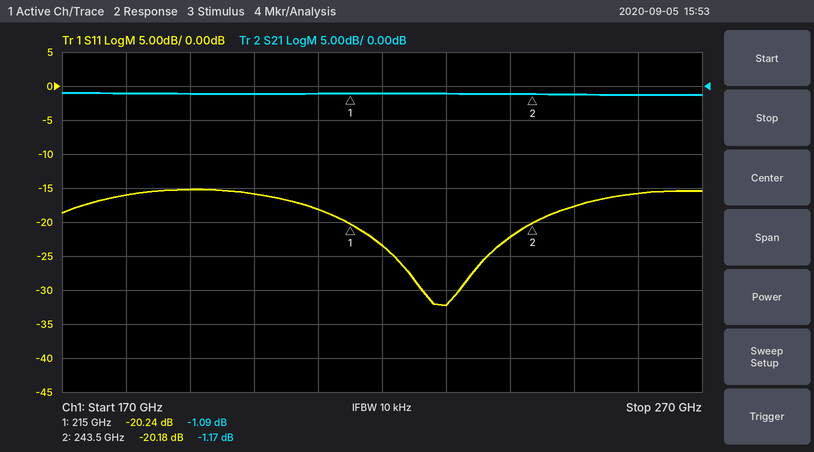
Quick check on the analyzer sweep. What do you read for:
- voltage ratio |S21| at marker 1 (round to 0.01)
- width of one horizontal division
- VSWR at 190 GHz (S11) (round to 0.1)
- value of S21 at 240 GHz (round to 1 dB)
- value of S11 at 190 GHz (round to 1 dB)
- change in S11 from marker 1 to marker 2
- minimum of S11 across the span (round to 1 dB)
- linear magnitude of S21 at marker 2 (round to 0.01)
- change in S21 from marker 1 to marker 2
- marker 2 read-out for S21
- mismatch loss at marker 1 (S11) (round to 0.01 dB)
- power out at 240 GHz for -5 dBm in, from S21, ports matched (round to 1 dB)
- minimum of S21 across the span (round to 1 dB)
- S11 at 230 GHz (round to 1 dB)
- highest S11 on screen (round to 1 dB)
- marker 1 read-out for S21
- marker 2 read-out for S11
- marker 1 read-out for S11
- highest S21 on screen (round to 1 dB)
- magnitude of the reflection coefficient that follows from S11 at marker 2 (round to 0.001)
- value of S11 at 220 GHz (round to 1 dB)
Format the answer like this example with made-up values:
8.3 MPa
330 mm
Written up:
0.88
10 GHz
1.4
-1 dB
-15 dB
0.06 dB
-32 dB
0.87
-0.08 dB
-1.17 dB
0.04 dB
-6 dBm
-1 dB
-32 dB
-15 dB
-1.09 dB
-20.18 dB
-20.24 dB
-1 dB
0.098
-23 dB
